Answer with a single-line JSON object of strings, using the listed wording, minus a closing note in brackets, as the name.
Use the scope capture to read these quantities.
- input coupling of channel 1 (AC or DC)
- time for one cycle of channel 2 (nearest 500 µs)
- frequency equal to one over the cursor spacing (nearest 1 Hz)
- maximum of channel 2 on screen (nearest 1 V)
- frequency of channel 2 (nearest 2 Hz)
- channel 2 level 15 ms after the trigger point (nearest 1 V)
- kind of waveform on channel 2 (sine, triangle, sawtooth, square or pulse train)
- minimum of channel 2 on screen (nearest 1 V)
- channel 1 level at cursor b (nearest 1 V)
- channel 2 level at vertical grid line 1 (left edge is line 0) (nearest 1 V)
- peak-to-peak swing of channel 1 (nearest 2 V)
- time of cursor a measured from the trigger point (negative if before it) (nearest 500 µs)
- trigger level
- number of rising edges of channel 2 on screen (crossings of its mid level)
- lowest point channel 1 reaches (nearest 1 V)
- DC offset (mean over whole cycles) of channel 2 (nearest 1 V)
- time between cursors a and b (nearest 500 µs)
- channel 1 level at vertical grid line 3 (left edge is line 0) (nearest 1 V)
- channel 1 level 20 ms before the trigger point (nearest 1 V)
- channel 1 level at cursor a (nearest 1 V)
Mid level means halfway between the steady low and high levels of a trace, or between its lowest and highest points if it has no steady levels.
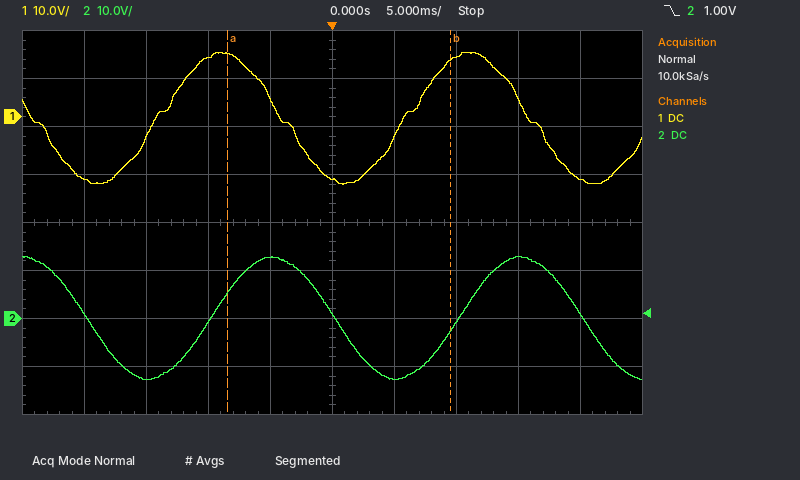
{"input coupling of channel 1": "DC", "time for one cycle of channel 2": "20.0 ms", "frequency equal to one over the cursor spacing": "56 Hz", "maximum of channel 2 on screen": "13 V", "frequency of channel 2": "50 Hz", "channel 2 level 15 ms after the trigger point": "13 V", "kind of waveform on channel 2": "sine", "minimum of channel 2 on screen": "-13 V", "channel 1 level at cursor b": "12 V", "channel 2 level at vertical grid line 1 (left edge is line 0)": "1 V", "peak-to-peak swing of channel 1": "28 V", "time of cursor a measured from the trigger point (negative if before it)": "-8.5 ms", "trigger level": "1.00 V", "number of rising edges of channel 2 on screen": "2", "lowest point channel 1 reaches": "-14 V", "DC offset (mean over whole cycles) of channel 2": "0 V", "time between cursors a and b": "18.0 ms", "channel 1 level at vertical grid line 3 (left edge is line 0)": "12 V", "channel 1 level 20 ms before the trigger point": "-13 V", "channel 1 level at cursor a": "13 V"}
